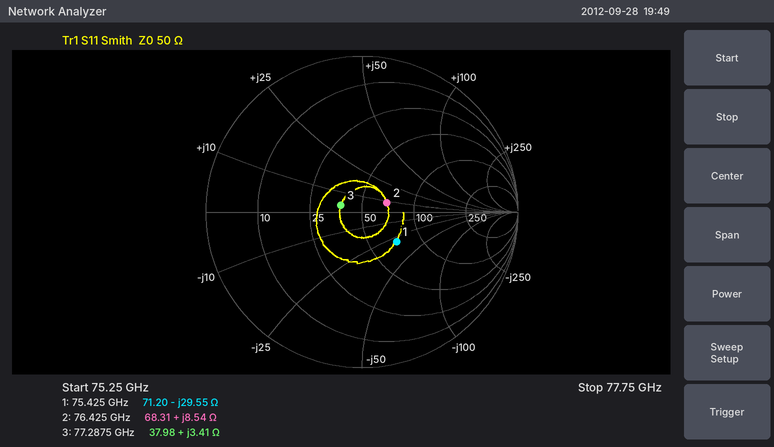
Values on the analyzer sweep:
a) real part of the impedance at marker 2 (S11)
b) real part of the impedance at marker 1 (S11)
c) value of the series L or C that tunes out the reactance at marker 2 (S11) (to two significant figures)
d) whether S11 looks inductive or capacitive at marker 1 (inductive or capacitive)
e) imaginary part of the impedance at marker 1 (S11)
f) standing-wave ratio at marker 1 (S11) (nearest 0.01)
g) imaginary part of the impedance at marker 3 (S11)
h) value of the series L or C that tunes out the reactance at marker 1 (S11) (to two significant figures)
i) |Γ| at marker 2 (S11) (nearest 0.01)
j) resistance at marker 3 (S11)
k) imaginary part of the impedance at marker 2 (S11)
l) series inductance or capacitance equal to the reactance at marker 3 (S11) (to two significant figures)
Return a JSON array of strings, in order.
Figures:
["68.31 Ω", "71.20 Ω", "240 fF", "capacitive", "-29.55 Ω", "1.82", "+3.41 Ω", "62 pH", "0.17", "37.98 Ω", "+8.54 Ω", "7.0 pH"]
